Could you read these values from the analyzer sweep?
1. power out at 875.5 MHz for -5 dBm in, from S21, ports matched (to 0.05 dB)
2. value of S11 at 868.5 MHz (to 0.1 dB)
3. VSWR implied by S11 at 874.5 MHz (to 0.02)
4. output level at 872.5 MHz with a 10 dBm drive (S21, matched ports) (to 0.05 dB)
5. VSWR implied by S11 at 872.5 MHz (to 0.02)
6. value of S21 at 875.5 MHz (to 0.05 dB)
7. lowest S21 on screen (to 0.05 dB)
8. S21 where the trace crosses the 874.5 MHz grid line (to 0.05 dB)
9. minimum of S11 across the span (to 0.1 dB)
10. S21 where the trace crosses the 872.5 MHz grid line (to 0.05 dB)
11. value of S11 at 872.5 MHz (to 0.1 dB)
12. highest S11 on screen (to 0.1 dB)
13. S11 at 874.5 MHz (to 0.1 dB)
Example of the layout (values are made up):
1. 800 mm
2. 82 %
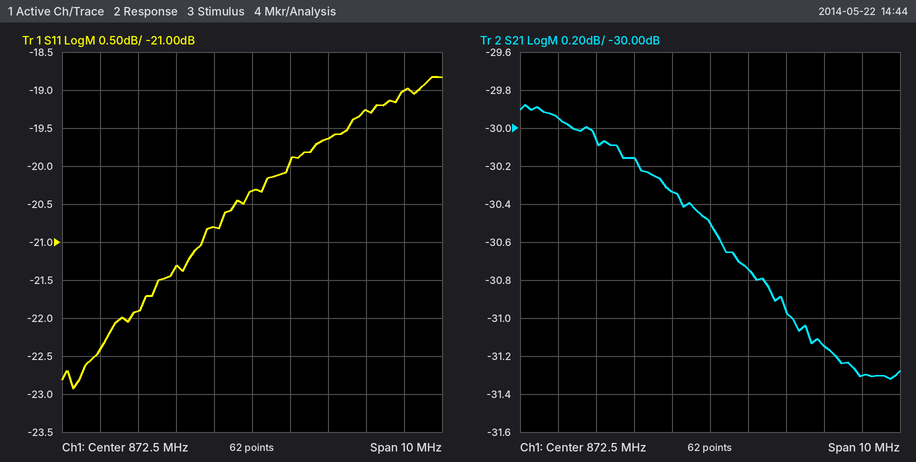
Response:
1. -36.15 dBm
2. -22.4 dB
3. 1.24
4. -20.50 dBm
5. 1.22
6. -31.15 dB
7. -31.30 dB
8. -30.95 dB
9. -22.9 dB
10. -30.50 dB
11. -20.3 dB
12. -18.8 dB
13. -19.6 dB
